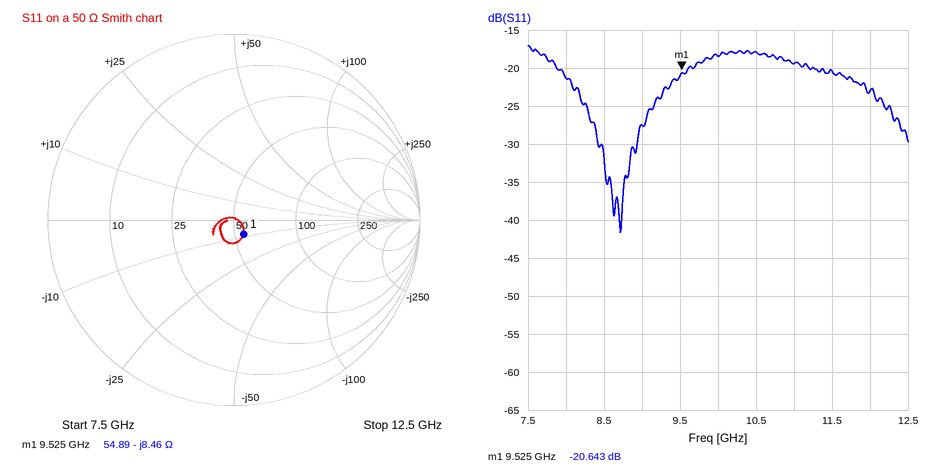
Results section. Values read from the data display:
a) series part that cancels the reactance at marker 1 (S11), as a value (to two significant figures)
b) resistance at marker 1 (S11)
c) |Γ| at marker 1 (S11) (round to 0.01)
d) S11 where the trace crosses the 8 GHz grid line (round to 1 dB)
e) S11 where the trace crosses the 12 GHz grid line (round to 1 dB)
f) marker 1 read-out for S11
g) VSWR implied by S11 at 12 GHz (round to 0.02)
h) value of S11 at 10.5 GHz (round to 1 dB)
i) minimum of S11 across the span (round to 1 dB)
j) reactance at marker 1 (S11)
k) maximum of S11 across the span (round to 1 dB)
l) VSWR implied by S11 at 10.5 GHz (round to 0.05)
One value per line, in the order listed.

140 pH
54.89 Ω
0.09
-21 dB
-23 dB
-20.643 dB
1.16
-18 dB
-42 dB
-8.46 Ω
-17 dB
1.30
